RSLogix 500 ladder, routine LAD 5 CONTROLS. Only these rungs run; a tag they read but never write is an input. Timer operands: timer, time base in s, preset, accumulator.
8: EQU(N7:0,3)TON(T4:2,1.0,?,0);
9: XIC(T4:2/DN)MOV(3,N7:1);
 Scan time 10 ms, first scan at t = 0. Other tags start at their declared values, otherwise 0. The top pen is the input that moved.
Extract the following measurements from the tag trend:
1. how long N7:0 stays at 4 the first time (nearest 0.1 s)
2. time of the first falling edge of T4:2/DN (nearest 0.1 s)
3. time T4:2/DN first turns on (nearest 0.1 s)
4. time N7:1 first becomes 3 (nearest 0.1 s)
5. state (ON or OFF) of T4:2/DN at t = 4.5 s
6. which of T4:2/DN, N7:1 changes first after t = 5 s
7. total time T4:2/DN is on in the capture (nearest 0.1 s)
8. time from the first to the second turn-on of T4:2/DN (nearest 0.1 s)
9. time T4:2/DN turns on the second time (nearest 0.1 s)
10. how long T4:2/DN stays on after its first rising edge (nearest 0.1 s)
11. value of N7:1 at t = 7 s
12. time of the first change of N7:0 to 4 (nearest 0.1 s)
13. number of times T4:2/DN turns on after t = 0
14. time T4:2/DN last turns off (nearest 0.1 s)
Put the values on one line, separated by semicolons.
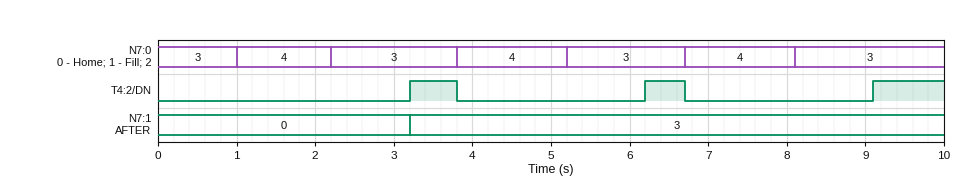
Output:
1.2 s; 3.8 s; 3.2 s; 3.2 s; OFF; T4:2/DN; 2.0 s; 3.0 s; 6.2 s; 0.6 s; 3; 1.0 s; 3; 6.7 s
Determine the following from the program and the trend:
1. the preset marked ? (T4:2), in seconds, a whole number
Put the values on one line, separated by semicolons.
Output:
1 s
